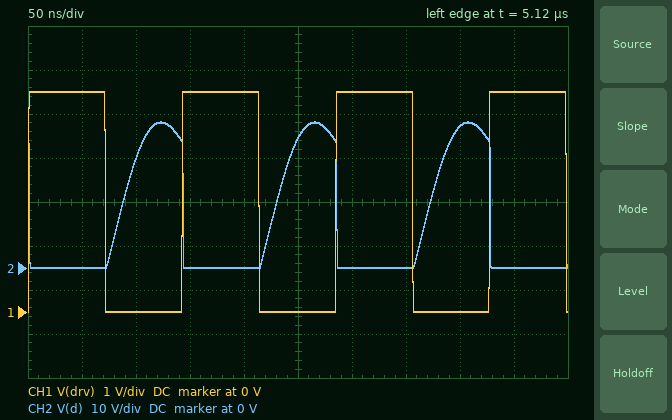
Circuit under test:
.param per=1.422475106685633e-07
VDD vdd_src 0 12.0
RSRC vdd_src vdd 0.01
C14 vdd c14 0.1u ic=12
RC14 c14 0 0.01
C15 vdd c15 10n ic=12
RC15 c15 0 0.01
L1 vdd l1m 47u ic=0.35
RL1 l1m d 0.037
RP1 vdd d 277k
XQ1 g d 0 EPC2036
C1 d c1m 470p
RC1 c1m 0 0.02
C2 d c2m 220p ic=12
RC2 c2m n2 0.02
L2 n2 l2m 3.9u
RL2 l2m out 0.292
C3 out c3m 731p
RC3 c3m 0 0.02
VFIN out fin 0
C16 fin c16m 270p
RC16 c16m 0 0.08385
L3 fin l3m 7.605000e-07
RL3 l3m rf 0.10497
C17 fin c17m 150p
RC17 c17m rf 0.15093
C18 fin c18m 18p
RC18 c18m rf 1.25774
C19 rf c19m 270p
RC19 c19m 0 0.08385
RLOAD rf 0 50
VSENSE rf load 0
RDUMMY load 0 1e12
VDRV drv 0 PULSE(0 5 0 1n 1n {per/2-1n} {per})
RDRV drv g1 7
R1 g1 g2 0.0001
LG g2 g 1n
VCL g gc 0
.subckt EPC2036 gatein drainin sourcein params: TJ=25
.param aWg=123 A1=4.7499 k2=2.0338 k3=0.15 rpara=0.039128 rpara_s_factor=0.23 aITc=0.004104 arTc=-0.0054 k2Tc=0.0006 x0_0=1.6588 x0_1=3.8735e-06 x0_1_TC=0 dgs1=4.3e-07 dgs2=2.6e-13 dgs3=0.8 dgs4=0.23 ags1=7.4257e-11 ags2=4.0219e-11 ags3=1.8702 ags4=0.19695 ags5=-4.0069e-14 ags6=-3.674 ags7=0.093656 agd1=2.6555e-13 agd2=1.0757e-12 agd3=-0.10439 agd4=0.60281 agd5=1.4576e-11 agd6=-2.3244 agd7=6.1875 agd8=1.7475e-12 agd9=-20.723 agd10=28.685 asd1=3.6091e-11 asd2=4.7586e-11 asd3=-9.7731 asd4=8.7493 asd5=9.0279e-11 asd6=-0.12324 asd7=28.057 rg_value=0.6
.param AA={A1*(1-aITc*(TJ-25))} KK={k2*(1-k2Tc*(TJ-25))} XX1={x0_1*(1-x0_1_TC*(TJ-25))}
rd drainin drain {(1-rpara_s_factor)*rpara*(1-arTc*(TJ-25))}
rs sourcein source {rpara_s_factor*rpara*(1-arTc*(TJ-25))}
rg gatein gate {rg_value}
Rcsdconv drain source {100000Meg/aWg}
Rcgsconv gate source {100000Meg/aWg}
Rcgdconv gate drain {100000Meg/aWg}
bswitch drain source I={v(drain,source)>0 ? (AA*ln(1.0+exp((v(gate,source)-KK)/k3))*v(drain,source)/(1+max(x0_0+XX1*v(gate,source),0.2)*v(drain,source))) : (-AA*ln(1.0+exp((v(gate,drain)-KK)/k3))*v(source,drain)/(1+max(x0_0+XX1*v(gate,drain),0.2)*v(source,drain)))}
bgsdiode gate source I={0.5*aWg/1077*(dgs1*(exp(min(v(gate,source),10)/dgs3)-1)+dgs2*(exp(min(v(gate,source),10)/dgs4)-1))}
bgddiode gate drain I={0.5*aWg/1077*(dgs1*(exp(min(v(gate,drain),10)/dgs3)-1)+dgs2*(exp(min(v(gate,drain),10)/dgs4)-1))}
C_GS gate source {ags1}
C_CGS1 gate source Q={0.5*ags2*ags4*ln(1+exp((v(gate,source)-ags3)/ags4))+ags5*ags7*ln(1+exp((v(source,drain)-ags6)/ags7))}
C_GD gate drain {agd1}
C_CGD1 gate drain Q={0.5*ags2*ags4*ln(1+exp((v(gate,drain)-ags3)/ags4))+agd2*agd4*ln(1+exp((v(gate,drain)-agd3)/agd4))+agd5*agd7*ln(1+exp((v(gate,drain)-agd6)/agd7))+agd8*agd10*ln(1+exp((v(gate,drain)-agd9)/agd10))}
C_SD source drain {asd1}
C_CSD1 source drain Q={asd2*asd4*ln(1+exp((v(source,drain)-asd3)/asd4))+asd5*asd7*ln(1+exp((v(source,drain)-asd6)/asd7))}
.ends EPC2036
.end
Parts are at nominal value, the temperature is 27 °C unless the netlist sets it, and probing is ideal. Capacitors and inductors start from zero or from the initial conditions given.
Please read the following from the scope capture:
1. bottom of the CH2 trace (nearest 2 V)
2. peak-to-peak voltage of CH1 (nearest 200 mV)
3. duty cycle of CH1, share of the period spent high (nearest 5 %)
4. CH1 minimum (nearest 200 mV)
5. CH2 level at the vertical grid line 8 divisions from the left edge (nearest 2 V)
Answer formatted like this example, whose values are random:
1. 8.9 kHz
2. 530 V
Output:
1. 0 V
2. 5.0 V
3. 50 %
4. 0 V
5. 32 V
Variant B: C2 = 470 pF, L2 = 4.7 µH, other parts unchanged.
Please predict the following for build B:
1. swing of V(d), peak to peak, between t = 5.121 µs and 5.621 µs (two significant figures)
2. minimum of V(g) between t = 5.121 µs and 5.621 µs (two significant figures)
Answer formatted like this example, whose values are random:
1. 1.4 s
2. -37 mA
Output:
1. 42 V
2. 1.4 mV
